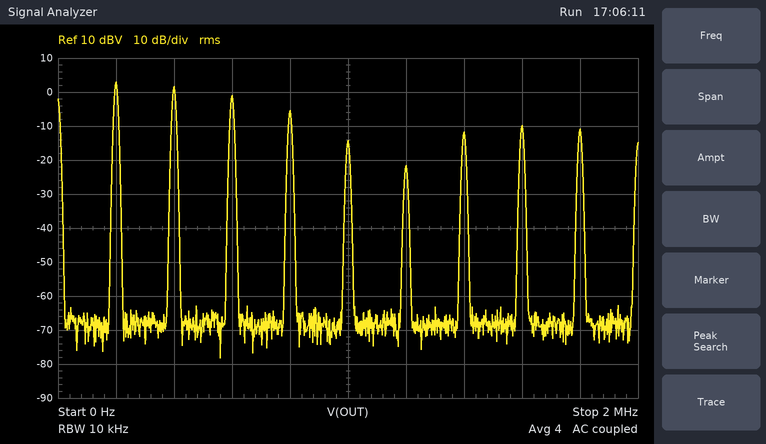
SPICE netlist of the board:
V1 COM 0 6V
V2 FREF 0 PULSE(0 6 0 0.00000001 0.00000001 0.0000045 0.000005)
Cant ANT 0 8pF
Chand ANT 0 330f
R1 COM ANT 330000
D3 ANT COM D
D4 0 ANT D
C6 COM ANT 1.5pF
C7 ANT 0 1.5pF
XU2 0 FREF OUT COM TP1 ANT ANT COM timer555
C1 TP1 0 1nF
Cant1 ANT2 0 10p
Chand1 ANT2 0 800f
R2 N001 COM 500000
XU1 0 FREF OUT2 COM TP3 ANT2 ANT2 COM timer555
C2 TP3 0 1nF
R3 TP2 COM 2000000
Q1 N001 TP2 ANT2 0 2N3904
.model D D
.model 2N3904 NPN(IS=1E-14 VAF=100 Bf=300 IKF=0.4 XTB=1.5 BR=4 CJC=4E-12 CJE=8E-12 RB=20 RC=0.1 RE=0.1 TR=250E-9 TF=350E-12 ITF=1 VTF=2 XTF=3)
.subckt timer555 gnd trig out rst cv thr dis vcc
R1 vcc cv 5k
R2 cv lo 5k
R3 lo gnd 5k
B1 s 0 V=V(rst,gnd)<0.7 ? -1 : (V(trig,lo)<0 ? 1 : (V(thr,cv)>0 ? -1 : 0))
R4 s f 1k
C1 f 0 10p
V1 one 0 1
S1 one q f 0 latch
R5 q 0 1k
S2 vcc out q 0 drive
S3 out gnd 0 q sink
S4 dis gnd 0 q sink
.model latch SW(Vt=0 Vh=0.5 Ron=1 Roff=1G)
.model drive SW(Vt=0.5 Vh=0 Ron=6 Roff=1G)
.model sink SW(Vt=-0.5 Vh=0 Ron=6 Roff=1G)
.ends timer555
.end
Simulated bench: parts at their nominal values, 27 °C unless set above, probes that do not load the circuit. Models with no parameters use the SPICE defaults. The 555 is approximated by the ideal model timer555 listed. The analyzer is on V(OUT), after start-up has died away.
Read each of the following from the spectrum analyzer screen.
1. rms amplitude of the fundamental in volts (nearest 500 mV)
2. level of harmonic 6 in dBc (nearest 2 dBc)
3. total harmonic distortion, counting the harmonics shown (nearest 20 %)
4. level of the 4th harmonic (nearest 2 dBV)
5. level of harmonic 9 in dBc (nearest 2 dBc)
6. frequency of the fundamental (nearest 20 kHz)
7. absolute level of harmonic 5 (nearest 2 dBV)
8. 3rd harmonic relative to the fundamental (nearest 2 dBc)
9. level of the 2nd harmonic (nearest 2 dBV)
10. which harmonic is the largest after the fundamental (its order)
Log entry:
1.5 V
-24 dBc
120 %
-6 dBV
-14 dBc
200 kHz
-14 dBV
-4 dBc
2 dBV
2
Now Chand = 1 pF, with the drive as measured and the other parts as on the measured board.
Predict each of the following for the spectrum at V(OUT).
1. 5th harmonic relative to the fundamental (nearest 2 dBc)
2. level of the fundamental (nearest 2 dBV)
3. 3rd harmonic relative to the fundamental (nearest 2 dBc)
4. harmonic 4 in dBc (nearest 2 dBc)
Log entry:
-6 dBc
0 dBV
-2 dBc
-4 dBc
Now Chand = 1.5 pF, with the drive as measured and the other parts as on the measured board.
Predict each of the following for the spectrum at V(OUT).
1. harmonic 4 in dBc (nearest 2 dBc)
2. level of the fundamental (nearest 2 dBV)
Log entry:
-2 dBc
-2 dBV
